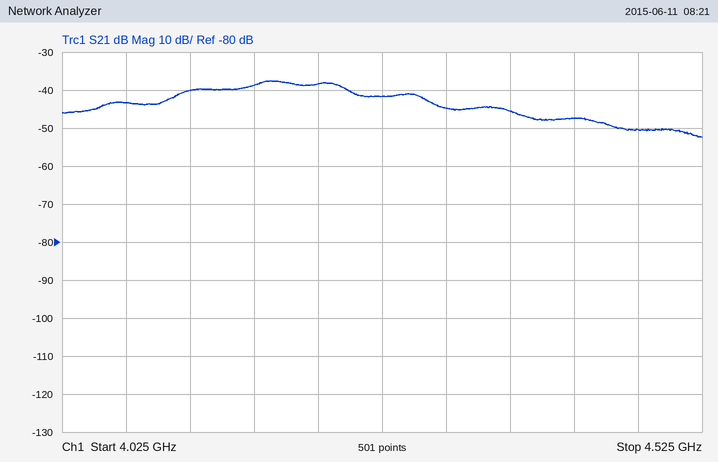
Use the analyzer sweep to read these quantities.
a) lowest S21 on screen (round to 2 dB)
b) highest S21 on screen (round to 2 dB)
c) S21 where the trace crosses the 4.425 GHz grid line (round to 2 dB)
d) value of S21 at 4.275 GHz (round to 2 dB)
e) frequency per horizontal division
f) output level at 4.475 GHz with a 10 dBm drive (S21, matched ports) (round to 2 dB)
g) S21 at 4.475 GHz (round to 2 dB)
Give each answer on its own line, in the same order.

-52 dB
-38 dB
-48 dB
-42 dB
50 MHz
-40 dBm
-50 dB
